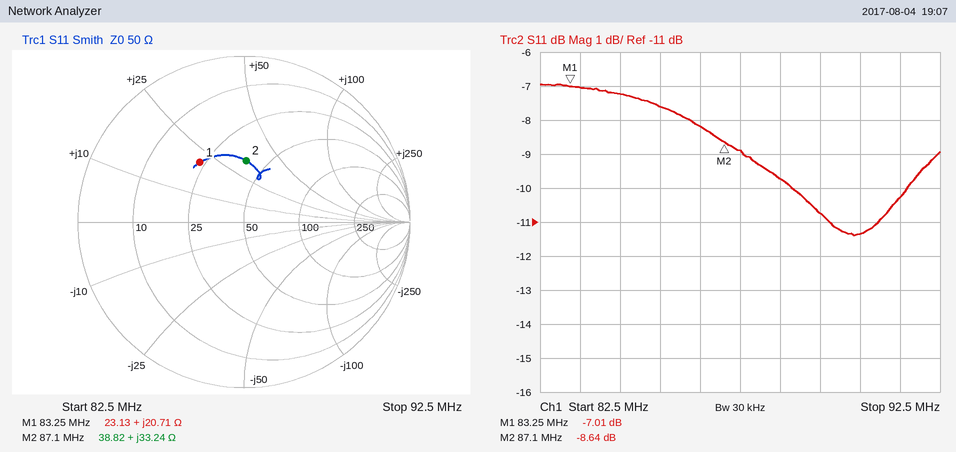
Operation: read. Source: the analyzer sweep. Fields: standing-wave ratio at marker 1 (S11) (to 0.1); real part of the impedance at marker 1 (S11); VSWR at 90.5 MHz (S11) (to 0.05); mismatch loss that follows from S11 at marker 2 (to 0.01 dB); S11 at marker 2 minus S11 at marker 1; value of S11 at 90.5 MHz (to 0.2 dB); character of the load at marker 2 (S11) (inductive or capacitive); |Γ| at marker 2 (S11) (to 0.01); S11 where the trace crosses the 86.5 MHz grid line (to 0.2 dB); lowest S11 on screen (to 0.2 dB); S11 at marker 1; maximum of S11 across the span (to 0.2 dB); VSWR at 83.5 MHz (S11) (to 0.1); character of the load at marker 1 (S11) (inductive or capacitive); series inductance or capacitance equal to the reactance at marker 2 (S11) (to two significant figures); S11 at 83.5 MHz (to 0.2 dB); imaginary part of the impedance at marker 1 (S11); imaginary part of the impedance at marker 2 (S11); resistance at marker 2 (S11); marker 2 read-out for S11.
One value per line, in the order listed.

2.6
23.13 Ω
1.75
0.64 dB
-1.63 dB
-11.4 dB
inductive
0.37
-8.2 dB
-11.4 dB
-7.01 dB
-7.0 dB
2.6
inductive
61 nH
-7.0 dB
+20.71 Ω
+33.24 Ω
38.82 Ω
-8.64 dB
